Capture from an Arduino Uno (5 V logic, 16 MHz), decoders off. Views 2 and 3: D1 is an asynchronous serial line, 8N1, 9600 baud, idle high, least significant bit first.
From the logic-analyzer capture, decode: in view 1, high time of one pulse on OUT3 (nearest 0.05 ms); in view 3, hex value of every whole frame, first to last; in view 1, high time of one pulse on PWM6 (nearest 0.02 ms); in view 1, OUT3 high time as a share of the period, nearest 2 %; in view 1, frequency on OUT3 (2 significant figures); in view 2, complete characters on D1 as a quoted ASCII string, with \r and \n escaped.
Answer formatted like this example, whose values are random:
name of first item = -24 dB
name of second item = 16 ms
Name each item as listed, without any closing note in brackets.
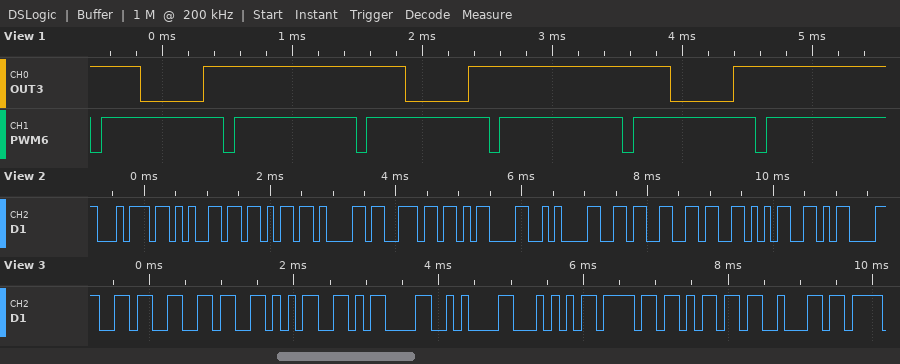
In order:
in view 1, high time of one pulse on OUT3 = 1.55 ms
in view 3, hex value of every whole frame, first to last = 36 36 35 0D 0A 54 6F 6D 62
in view 1, high time of one pulse on PWM6 = 0.94 ms
in view 1, OUT3 high time as a share of the period, nearest 2 % = 76 %
in view 1, frequency on OUT3 = 490 Hz
in view 2, complete characters on D1 as a quoted ASCII string, with \r and \n escaped = "tekan\r\n665\r"
